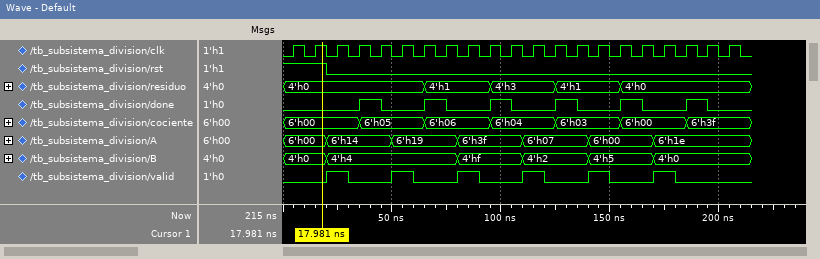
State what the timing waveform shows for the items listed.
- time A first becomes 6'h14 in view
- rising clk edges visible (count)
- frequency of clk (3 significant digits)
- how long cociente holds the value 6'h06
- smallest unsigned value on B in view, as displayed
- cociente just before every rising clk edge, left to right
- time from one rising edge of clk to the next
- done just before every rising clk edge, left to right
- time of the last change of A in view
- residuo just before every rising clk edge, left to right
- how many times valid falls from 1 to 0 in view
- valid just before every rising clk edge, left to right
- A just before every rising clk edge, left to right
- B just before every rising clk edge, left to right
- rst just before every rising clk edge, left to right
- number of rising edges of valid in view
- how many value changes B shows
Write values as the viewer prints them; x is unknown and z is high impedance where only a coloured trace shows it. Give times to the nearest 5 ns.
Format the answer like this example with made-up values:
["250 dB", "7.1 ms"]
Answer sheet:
["20 ns", "21", "100 MHz", "30 ns", "4'h0", "6'h00, 6'h00, 6'h00, 6'h00, 6'h05, 6'h05, 6'h05, 6'h06, 6'h06, 6'h06, 6'h04, 6'h04, 6'h04, 6'h03, 6'h03, 6'h03, 6'h00, 6'h00, 6'h00, 6'h3f, 6'h3f", "10 ns", "0 0 0 0 1 0 0 1 0 0 1 0 0 1 0 0 1 0 0 1 0", "170 ns", "4'h0, 4'h0, 4'h0, 4'h0, 4'h0, 4'h0, 4'h0, 4'h1, 4'h1, 4'h1, 4'h3, 4'h3, 4'h3, 4'h1, 4'h1, 4'h1, 4'h0, 4'h0, 4'h0, 4'h0, 4'h0", "6", "0 0 1 0 0 1 0 0 1 0 0 1 0 0 1 0 0 1 0 0 0", "6'h00, 6'h00, 6'h14, 6'h14, 6'h14, 6'h19, 6'h19, 6'h19, 6'h3f, 6'h3f, 6'h3f, 6'h07, 6'h07, 6'h07, 6'h00, 6'h00, 6'h00, 6'h1e, 6'h1e, 6'h1e, 6'h1e", "4'h0, 4'h0, 4'h4, 4'h4, 4'h4, 4'h4, 4'h4, 4'h4, 4'hf, 4'hf, 4'hf, 4'h2, 4'h2, 4'h2, 4'h5, 4'h5, 4'h5, 4'h0, 4'h0, 4'h0, 4'h0", "1 1 0 0 0 0 0 0 0 0 0 0 0 0 0 0 0 0 0 0 0", "6", "5"]
